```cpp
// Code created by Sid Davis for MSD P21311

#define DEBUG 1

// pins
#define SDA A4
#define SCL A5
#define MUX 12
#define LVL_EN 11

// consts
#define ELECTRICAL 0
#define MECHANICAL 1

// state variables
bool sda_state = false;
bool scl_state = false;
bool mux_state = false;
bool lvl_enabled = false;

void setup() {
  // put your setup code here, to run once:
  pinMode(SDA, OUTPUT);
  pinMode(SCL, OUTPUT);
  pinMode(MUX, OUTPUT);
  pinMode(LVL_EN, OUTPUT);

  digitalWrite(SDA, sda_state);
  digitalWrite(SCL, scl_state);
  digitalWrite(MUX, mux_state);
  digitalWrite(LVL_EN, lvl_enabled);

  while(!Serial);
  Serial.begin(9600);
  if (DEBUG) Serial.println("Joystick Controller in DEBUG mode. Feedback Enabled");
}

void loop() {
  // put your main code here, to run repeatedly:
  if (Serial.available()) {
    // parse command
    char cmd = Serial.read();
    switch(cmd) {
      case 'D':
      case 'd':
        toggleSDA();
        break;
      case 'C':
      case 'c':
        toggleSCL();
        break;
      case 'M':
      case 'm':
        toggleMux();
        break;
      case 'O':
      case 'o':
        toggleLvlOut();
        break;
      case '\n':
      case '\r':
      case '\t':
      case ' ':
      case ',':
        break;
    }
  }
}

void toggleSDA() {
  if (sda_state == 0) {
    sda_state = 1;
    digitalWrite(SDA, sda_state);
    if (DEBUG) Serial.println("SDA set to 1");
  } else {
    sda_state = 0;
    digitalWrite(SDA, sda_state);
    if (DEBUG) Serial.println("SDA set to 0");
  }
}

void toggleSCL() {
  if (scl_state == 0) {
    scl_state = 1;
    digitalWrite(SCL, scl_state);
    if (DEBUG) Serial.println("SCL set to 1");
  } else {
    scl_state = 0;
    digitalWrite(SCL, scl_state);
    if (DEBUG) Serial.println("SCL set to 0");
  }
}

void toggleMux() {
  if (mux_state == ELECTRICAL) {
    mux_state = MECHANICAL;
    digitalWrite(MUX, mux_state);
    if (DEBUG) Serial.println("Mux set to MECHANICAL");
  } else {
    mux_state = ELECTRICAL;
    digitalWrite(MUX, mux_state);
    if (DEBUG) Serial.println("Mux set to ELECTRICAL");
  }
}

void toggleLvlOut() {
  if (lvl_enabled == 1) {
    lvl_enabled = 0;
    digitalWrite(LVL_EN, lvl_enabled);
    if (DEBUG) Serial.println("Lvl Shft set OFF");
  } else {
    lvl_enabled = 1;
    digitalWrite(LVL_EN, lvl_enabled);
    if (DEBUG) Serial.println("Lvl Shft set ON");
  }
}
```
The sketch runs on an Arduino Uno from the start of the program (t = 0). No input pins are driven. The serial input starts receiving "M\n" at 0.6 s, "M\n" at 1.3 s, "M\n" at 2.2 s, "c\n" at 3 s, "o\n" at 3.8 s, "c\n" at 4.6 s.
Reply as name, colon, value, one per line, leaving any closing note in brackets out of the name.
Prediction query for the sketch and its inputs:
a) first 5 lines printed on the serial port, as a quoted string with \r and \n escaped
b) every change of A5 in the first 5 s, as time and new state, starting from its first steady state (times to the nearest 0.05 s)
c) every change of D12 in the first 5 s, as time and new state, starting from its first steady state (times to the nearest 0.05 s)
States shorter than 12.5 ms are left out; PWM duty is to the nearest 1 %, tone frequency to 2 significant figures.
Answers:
first 5 lines printed on the serial port, as a quoted string with \r and \n escaped: "Joystick Controller in DEBUG mode. Feedback Enabled\r\nMux set to MECHANICAL\r\nMux set to ELECTRICAL\r\nMux set to MECHANICAL\r\nSCL set to 1\r\n"
every change of A5 in the first 5 s, as time and new state, starting from its first steady state: 0 s low; 3 s high; 4.6 s low
every change of D12 in the first 5 s, as time and new state, starting from its first steady state: 0 s low; 0.6 s high; 1.3 s low; 2.2 s high
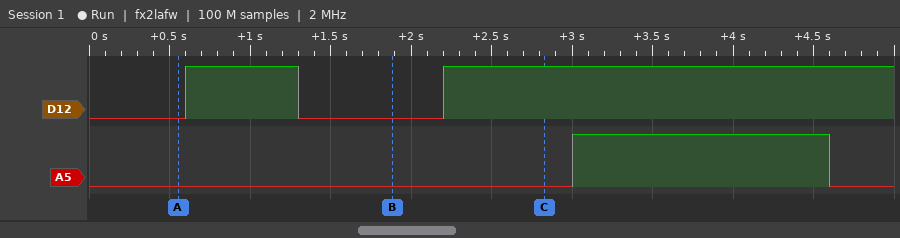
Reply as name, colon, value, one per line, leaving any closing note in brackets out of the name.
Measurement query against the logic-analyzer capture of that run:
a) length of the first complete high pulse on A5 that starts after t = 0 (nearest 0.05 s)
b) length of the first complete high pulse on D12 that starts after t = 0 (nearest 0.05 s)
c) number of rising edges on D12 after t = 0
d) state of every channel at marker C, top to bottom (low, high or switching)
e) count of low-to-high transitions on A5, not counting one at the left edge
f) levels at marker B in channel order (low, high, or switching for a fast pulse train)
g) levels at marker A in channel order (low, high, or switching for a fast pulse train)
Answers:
length of the first complete high pulse on A5 that starts after t = 0: 1.60 s
length of the first complete high pulse on D12 that starts after t = 0: 0.70 s
number of rising edges on D12 after t = 0: 2
state of every channel at marker C, top to bottom: D12 high, A5 low
count of low-to-high transitions on A5, not counting one at the left edge: 1
levels at marker B in channel order: D12 low, A5 low
levels at marker A in channel order: D12 low, A5 low
